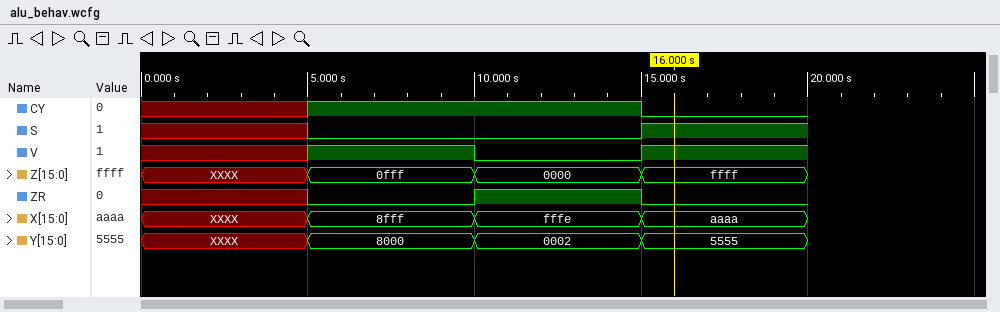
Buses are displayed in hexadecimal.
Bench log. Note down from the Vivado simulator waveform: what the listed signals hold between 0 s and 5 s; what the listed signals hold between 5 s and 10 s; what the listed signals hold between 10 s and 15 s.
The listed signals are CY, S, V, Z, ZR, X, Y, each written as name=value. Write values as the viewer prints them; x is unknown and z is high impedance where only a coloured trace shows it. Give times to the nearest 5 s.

CY=x, S=x, V=x, Z=XXXX, ZR=x, X=XXXX, Y=XXXX
CY=1, S=0, V=1, Z=0fff, ZR=0, X=8fff, Y=8000
CY=1, S=0, V=0, Z=0000, ZR=1, X=fffe, Y=0002
